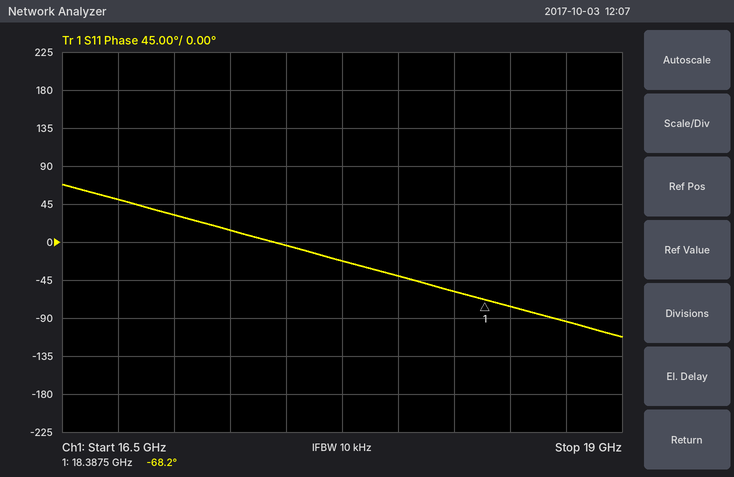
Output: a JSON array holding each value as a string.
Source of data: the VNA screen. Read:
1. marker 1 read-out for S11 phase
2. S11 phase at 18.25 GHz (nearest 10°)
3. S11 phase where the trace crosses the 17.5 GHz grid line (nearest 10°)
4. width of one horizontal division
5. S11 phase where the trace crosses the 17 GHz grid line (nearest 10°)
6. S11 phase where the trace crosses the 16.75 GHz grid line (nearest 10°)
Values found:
["-68.2°", "-60°", "0°", "250 MHz", "30°", "50°"]
